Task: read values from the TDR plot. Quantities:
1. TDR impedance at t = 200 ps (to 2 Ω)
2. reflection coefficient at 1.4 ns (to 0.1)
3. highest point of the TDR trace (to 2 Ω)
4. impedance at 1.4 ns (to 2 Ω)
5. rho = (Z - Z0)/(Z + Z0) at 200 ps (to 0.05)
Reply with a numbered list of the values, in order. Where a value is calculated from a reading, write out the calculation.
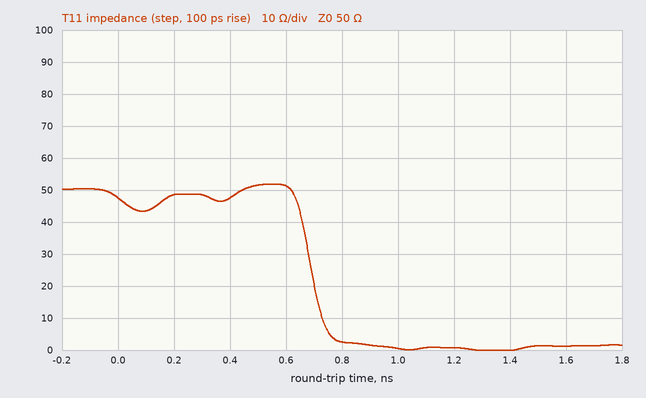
1. 48 Ω
2. (0 − 50)/(0 + 50) ≈ -1.0
3. 52 Ω
4. 0 Ω
5. (48 − 50)/(48 + 50) ≈ 0.00
